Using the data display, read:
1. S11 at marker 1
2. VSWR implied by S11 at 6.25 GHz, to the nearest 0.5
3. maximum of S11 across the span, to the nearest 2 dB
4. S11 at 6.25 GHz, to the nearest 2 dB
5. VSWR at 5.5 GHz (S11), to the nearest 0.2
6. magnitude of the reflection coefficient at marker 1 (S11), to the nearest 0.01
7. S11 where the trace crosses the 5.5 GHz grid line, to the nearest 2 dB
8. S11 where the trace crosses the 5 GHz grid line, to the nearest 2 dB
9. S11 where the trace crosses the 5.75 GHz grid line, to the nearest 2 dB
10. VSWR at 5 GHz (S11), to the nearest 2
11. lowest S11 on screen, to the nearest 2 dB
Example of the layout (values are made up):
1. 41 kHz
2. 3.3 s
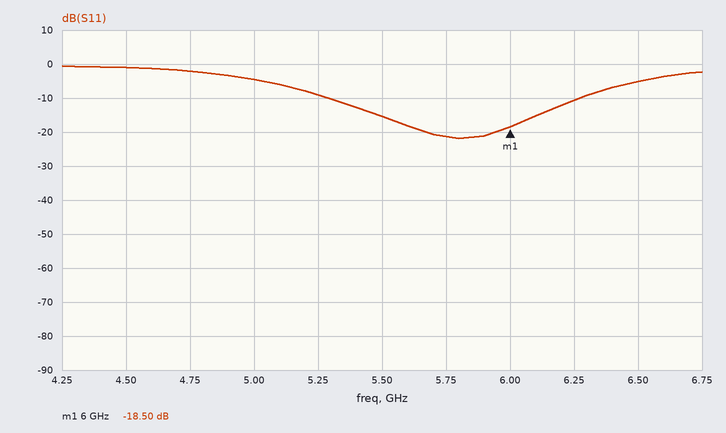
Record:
1. -18.50 dB
2. 2.0
3. 0 dB
4. -10 dB
5. 1.4
6. 0.12
7. -16 dB
8. -4 dB
9. -22 dB
10. 4
11. -22 dB
